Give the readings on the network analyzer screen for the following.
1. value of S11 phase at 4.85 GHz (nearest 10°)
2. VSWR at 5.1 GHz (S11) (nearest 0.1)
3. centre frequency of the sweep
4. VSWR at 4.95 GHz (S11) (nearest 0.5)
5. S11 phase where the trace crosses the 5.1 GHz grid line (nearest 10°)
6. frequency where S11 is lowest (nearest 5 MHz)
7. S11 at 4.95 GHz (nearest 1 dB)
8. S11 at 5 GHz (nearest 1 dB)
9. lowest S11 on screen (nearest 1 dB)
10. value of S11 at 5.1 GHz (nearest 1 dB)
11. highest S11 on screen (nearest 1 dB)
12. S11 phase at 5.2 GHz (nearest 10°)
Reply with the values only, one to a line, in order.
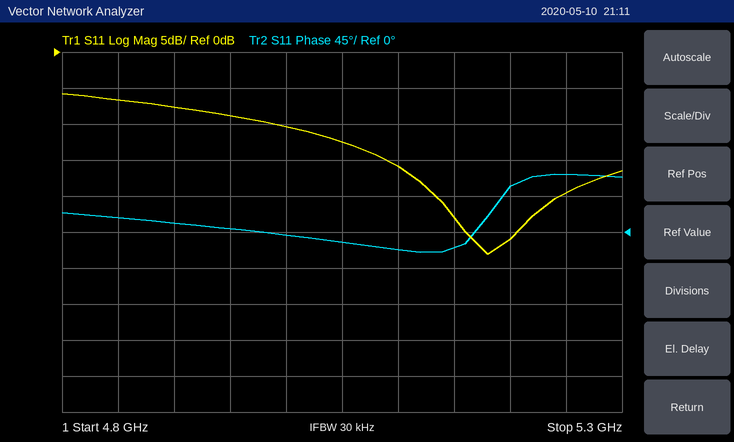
20°
1.4
5.05 GHz
2.0
-20°
5.180 GHz
-9 dB
-10 dB
-28 dB
-16 dB
-6 dB
60°
